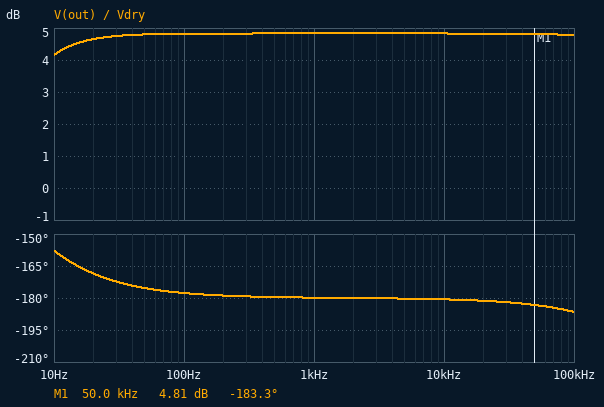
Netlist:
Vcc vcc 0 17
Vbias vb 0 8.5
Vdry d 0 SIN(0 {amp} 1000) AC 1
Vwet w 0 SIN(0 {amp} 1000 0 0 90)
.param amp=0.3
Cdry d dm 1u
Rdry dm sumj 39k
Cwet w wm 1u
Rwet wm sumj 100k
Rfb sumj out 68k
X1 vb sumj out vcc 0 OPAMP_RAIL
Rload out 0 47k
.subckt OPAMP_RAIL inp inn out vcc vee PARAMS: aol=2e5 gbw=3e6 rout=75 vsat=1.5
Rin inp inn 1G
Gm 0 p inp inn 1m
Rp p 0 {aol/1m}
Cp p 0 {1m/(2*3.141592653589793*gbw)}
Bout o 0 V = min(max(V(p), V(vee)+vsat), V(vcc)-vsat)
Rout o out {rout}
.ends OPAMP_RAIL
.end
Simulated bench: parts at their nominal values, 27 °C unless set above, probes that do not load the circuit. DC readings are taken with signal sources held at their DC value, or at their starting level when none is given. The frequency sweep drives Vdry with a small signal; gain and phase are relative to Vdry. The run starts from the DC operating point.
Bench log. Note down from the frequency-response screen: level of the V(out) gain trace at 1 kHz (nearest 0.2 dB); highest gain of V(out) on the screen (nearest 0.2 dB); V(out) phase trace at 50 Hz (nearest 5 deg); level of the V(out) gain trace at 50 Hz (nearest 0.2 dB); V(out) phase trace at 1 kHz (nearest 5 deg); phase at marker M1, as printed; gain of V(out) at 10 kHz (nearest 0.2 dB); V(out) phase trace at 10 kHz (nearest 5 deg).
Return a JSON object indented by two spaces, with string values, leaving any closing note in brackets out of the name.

{
  "level of the V(out) gain trace at 1 kHz": "4.8 dB",
  "highest gain of V(out) on the screen": "4.8 dB",
  "V(out) phase trace at 50 Hz": "-175 deg",
  "level of the V(out) gain trace at 50 Hz": "4.8 dB",
  "V(out) phase trace at 1 kHz": "-180 deg",
  "phase at marker M1, as printed": "-183.3 deg",
  "gain of V(out) at 10 kHz": "4.8 dB",
  "V(out) phase trace at 10 kHz": "-180 deg"
}
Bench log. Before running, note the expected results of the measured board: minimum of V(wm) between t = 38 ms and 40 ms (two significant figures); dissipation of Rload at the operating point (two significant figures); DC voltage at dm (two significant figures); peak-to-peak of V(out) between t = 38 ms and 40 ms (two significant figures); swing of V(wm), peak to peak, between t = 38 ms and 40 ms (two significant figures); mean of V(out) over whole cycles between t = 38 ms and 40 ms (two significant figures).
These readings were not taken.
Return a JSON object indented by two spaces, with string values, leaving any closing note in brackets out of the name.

{
  "minimum of V(wm) between t = 38 ms and 40 ms": "8.0 V",
  "dissipation of Rload at the operating point": "1.5 mW",
  "DC voltage at dm": "8.5 V",
  "peak-to-peak of V(out) between t = 38 ms and 40 ms": "1.1 V",
  "swing of V(wm), peak to peak, between t = 38 ms and 40 ms": "600 mV",
  "mean of V(out) over whole cycles between t = 38 ms and 40 ms": "8.6 V"
}
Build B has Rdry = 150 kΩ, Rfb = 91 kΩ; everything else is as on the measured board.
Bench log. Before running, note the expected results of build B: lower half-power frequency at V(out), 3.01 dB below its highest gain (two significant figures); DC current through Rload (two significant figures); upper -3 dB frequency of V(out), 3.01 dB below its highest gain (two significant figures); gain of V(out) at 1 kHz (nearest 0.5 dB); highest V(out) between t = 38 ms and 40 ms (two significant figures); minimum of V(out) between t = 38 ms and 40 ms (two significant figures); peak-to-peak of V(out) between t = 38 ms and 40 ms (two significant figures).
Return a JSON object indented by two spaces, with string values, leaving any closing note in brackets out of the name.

{
  "lower half-power frequency at V(out), 3.01 dB below its highest gain": "1.1 Hz",
  "DC current through Rload": "180 µA",
  "upper -3 dB frequency of V(out), 3.01 dB below its highest gain": "1.2 MHz",
  "gain of V(out) at 1 kHz": "-4.5 dB",
  "highest V(out) between t = 38 ms and 40 ms": "9.0 V",
  "minimum of V(out) between t = 38 ms and 40 ms": "8.4 V",
  "peak-to-peak of V(out) between t = 38 ms and 40 ms": "660 mV"
}
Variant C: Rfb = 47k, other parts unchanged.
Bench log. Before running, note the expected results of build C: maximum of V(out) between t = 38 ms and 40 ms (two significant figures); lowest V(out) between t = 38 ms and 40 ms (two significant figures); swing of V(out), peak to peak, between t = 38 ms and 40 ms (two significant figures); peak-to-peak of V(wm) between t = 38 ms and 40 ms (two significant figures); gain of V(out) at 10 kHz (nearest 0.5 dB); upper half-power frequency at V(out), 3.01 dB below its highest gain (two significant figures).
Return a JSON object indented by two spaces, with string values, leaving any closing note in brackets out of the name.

{
  "maximum of V(out) between t = 38 ms and 40 ms": "9.0 V",
  "lowest V(out) between t = 38 ms and 40 ms": "8.2 V",
  "swing of V(out), peak to peak, between t = 38 ms and 40 ms": "780 mV",
  "peak-to-peak of V(wm) between t = 38 ms and 40 ms": "600 mV",
  "gain of V(out) at 10 kHz": "1.5 dB",
  "upper half-power frequency at V(out), 3.01 dB below its highest gain": "1.1 MHz"
}
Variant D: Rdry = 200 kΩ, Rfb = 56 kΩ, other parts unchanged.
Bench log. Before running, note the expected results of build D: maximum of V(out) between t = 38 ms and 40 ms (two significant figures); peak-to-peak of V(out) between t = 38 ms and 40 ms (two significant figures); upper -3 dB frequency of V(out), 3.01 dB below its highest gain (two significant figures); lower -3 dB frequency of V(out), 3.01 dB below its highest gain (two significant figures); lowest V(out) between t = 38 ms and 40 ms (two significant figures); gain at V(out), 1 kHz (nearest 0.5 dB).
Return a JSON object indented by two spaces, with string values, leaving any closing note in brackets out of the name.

{
  "maximum of V(out) between t = 38 ms and 40 ms": "8.8 V",
  "peak-to-peak of V(out) between t = 38 ms and 40 ms": "380 mV",
  "upper -3 dB frequency of V(out), 3.01 dB below its highest gain": "1.6 MHz",
  "lower -3 dB frequency of V(out), 3.01 dB below its highest gain": "800 mHz",
  "lowest V(out) between t = 38 ms and 40 ms": "8.4 V",
  "gain at V(out), 1 kHz": "-11.0 dB"
}
